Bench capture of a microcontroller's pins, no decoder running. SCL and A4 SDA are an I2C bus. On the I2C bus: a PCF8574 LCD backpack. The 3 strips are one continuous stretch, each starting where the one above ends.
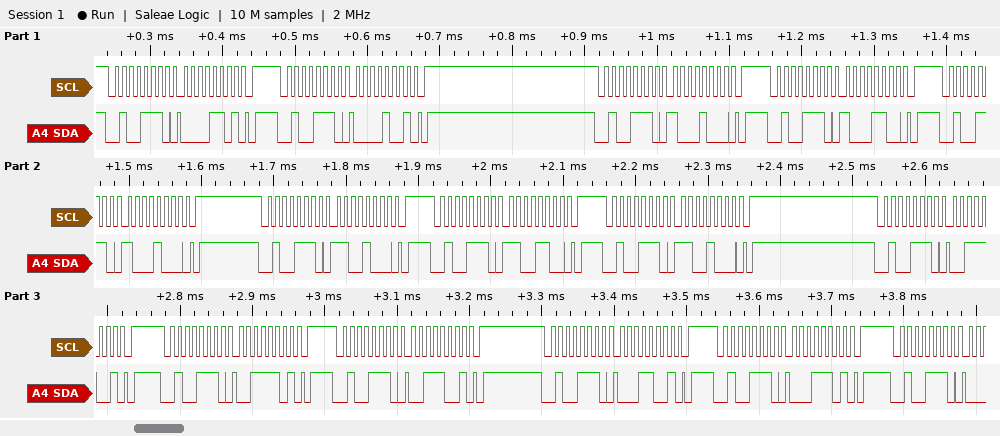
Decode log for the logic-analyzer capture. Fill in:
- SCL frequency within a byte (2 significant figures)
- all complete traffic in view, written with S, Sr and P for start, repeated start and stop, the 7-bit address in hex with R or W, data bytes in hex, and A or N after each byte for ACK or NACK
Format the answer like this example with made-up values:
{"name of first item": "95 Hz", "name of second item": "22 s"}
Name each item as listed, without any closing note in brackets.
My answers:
{"SCL frequency within a byte": "100 kHz", "all complete traffic in view, written with S, Sr and P for start, repeated start and stop, the 7-bit address in hex with R or W, data bytes in hex, and A or N after each byte for ACK or NACK": "S 27W A 0D A P S 27W A 09 A P S 27W A 88 A P S 27W A 8C A P S 27W A 88 A P S 27W A C8 A P S 27W A CC A P S 27W A C8 A P S 27W A 39 A P S 27W A 3D A P S 27W A 39 A P S 27W A 19 A P S 27W A 1D A P S 27W A"}
